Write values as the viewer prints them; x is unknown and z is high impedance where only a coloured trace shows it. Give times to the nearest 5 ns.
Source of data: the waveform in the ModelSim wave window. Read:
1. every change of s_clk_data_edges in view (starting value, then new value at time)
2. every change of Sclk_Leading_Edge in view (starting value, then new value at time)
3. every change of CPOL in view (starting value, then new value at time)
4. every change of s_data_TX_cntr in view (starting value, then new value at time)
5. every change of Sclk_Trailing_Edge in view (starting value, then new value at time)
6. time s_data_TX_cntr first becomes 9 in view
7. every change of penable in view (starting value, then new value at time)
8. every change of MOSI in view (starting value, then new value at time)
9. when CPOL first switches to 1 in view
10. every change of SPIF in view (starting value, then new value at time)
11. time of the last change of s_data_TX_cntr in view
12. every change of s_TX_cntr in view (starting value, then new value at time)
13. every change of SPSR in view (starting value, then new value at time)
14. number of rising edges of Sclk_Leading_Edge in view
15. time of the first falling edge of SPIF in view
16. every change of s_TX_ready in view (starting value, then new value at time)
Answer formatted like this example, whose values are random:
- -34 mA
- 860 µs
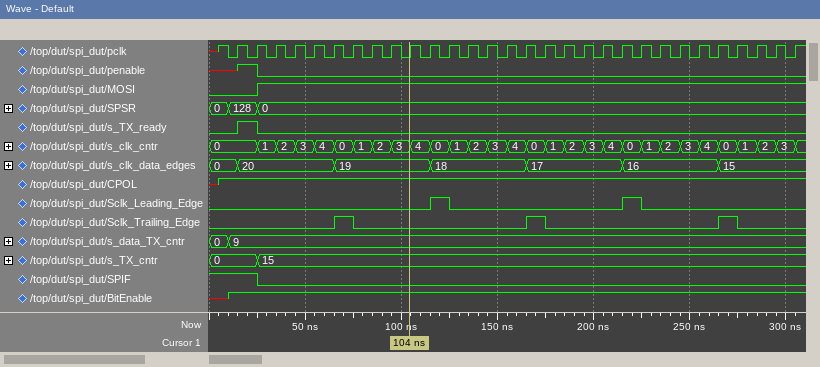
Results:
- 0, 20 at 15 ns, 19 at 65 ns, 18 at 115 ns, 17 at 165 ns, 16 at 215 ns, 15 at 265 ns
- 0, 1 at 115 ns, 0 at 125 ns, 1 at 215 ns, 0 at 225 ns
- x, 1 at 5 ns
- 0, 9 at 10 ns
- 0, 1 at 65 ns, 0 at 75 ns, 1 at 165 ns, 0 at 175 ns, 1 at 265 ns, 0 at 275 ns
- 10 ns
- x, 1 at 15 ns, 0 at 25 ns
- 0, 1 at 25 ns
- 5 ns
- 1, 0 at 25 ns
- 10 ns
- 0, 15 at 25 ns
- 0, 128 at 10 ns, 0 at 25 ns
- 2
- 25 ns
- 0, 1 at 15 ns, 0 at 25 ns
